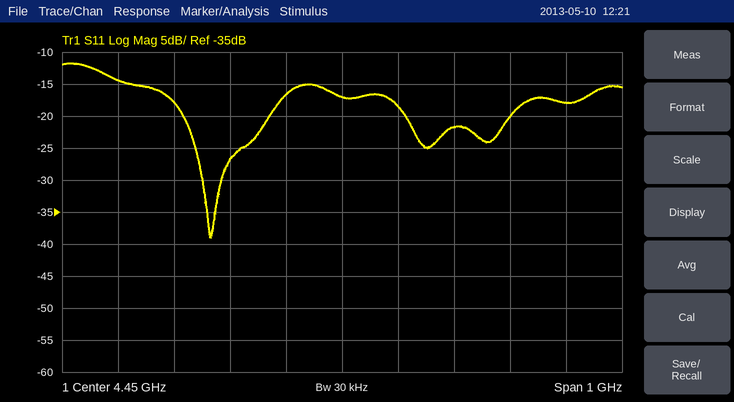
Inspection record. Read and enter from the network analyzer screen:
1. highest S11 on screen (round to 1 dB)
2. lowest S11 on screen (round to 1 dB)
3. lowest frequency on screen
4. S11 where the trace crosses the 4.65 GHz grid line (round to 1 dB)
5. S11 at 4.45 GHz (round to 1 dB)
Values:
-12 dB
-39 dB
3.95 GHz
-22 dB
-17 dB
